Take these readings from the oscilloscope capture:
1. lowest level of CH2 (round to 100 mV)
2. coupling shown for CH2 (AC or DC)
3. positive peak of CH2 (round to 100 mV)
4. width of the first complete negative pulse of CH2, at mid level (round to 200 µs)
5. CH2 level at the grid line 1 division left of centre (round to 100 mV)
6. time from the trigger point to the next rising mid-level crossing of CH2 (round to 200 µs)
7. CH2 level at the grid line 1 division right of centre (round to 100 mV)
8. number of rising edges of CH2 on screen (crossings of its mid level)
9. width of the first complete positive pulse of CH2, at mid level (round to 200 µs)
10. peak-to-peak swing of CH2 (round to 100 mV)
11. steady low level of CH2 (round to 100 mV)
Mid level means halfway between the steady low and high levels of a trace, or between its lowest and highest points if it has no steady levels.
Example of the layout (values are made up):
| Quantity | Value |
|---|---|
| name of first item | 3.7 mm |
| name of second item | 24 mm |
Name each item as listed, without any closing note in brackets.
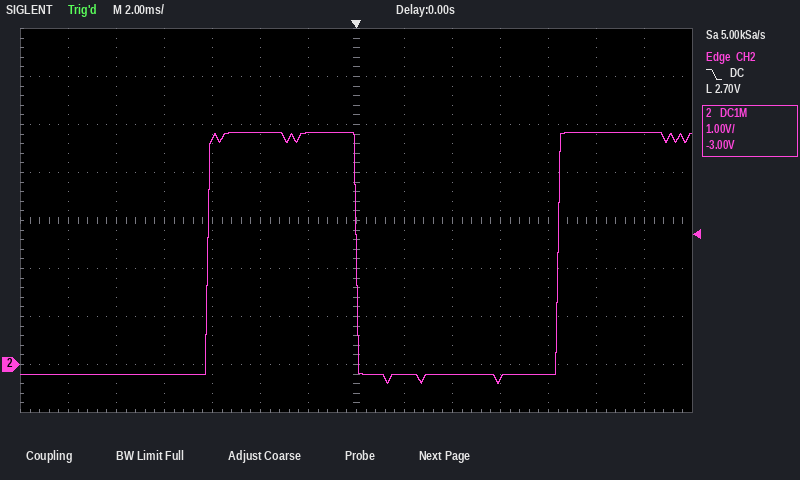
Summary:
| Quantity | Value |
|---|---|
| lowest level of CH2 | -400 mV |
| coupling shown for CH2 | DC |
| positive peak of CH2 | 4.8 V |
| width of the first complete negative pulse of CH2, at mid level | 8.4 ms |
| CH2 level at the grid line 1 division left of centre | 4.8 V |
| time from the trigger point to the next rising mid-level crossing of CH2 | 8.4 ms |
| CH2 level at the grid line 1 division right of centre | -200 mV |
| number of rising edges of CH2 on screen | 2 |
| width of the first complete positive pulse of CH2, at mid level | 6.2 ms |
| peak-to-peak swing of CH2 | 5.2 V |
| steady low level of CH2 | -200 mV |
